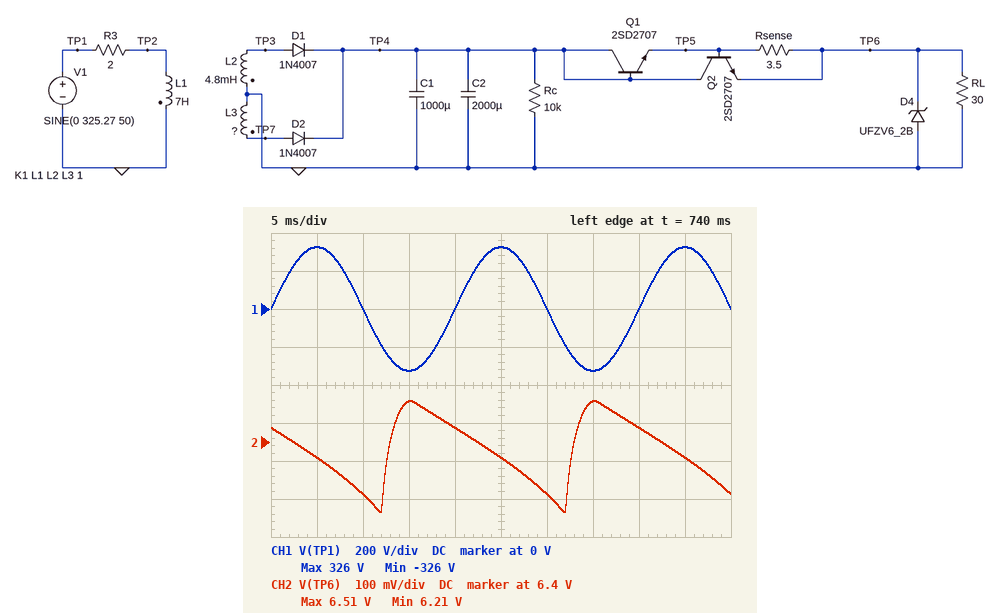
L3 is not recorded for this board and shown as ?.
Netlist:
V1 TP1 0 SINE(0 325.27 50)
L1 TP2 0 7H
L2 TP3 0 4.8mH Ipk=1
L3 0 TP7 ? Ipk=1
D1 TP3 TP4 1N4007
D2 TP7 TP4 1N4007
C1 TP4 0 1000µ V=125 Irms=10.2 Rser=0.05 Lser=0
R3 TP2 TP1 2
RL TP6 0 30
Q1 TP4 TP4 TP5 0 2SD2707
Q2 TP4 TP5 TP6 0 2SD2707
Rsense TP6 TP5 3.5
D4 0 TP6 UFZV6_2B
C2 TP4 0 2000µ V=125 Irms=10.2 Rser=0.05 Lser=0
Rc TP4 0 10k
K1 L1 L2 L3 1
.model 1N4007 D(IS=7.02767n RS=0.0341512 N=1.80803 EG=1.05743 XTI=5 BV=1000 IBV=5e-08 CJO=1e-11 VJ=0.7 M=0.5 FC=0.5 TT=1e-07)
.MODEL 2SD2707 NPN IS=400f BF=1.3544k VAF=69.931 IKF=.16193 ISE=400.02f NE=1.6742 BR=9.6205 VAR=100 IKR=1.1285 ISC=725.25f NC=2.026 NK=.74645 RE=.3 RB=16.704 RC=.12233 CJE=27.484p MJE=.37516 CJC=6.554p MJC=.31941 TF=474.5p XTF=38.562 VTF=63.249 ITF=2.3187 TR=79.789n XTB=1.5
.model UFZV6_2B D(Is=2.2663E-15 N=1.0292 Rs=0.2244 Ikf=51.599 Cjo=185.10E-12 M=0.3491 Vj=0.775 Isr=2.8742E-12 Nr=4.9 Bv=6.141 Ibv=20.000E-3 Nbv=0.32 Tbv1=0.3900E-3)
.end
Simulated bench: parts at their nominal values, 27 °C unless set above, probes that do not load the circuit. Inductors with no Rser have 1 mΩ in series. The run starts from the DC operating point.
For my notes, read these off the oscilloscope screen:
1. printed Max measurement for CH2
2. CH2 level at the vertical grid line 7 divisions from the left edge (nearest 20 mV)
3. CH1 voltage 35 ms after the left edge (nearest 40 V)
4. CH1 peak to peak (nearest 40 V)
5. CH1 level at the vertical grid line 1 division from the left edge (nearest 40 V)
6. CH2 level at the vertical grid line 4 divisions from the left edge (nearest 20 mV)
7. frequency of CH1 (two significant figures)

6.51 V
6.50 V
-320 V
640 V
320 V
6.44 V
50 Hz
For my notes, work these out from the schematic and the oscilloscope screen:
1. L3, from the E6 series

15 mH
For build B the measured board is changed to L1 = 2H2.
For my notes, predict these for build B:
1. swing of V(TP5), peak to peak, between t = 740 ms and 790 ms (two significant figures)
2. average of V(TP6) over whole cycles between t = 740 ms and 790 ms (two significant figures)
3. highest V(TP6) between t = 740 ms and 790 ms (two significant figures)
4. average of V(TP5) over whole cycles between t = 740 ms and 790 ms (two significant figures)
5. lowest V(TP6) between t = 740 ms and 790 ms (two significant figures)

3.1 V
6.6 V
6.8 V
11 V
6.5 V
